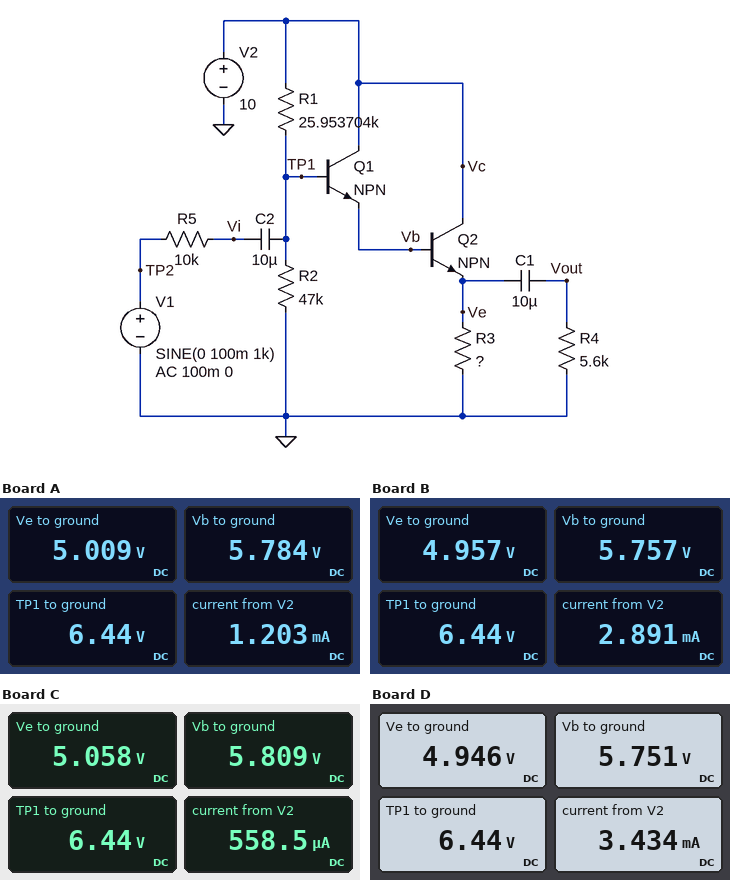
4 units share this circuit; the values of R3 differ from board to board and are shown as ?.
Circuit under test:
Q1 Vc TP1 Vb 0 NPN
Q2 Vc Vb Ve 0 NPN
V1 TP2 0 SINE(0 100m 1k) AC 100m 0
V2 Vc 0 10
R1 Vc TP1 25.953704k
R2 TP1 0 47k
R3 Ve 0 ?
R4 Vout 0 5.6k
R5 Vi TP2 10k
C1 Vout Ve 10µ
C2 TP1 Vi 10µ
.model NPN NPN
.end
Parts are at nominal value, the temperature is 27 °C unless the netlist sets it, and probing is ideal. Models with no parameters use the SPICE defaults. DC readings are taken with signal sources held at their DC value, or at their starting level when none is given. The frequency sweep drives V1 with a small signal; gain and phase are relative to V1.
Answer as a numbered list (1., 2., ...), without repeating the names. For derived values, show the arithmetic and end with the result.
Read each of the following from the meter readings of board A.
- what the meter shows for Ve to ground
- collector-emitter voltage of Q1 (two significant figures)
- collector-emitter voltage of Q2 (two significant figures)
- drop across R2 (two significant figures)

1. 5.009 V
2. 10 V - 5.784 V = 4.2 V
3. 10 V - 5.009 V = 5.0 V
4. 6.44 V = 6.4 V
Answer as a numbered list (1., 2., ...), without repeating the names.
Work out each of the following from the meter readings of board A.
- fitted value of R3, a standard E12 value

1. 4.7 kΩ
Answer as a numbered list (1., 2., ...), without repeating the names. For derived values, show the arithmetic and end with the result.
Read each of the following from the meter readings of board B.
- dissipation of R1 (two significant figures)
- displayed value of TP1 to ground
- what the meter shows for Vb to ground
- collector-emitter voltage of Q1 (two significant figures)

1. (10 V - 6.44 V)^2 / 25.95 kΩ = 490 µW
2. 6.44 V
3. 5.757 V
4. 10 V - 5.757 V = 4.2 V
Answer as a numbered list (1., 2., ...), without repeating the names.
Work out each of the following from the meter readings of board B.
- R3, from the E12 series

1. 1.8 kΩ
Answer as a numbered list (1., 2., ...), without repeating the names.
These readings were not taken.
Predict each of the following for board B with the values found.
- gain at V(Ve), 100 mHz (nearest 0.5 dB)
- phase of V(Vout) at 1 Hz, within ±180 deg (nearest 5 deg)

1. -20.0 dB
2. 100 deg
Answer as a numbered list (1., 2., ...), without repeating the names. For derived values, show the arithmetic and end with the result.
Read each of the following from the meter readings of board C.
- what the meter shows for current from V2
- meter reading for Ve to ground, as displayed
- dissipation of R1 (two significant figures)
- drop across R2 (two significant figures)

1. 558.5 µA
2. 5.058 V
3. (10 V - 6.44 V)^2 / 25.95 kΩ = 490 µW
4. 6.44 V = 6.4 V
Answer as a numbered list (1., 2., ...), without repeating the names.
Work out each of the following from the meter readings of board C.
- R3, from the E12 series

1. 12 kΩ
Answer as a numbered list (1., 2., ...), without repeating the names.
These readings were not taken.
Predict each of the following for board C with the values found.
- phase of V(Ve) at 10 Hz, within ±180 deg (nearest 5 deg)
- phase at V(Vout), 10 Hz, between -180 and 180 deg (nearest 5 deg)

1. 5 deg
2. 20 deg
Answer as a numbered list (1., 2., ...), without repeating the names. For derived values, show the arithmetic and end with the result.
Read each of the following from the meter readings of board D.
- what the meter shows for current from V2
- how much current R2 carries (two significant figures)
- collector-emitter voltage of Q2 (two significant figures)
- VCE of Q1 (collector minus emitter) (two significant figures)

1. 3.434 mA
2. (6.44 V) / 47 kΩ = 140 µA
3. 10 V - 4.946 V = 5.1 V
4. 10 V - 5.751 V = 4.2 V
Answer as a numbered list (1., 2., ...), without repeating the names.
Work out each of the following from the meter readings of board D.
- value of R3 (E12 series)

1. 1.5 kΩ
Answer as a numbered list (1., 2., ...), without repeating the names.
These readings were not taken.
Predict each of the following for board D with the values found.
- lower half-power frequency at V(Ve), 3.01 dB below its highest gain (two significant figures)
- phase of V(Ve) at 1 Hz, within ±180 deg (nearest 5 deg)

1. 590 mHz
2. 30 deg
